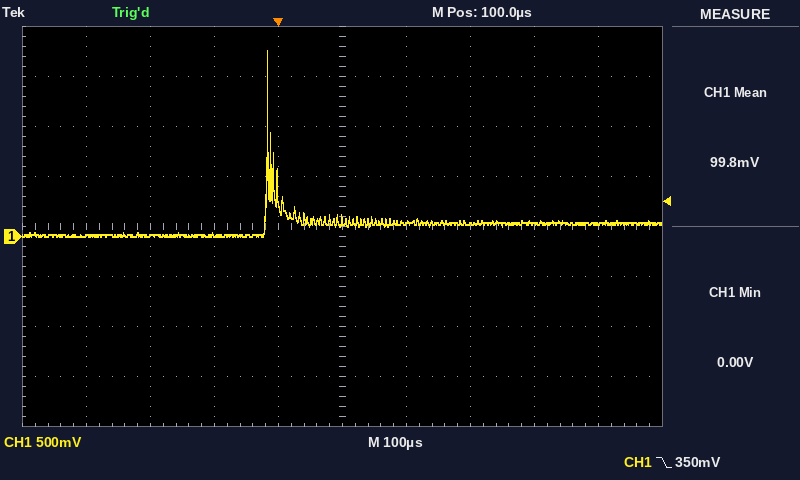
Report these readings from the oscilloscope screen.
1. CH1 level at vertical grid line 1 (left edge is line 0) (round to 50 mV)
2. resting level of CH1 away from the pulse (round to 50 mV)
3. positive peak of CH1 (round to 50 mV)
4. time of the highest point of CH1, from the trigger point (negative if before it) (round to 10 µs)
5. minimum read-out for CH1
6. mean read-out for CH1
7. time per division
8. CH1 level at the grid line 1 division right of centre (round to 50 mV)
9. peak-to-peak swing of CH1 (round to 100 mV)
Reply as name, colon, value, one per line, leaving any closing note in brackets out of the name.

CH1 level at vertical grid line 1 (left edge is line 0): 0 mV
resting level of CH1 away from the pulse: 150 mV
positive peak of CH1: 1.85 V
time of the highest point of CH1, from the trigger point (negative if before it): -20 µs
minimum read-out for CH1: 0.00 V
mean read-out for CH1: 99.8 mV
time per division: 100 µs
CH1 level at the grid line 1 division right of centre: 150 mV
peak-to-peak swing of CH1: 1.90 V
